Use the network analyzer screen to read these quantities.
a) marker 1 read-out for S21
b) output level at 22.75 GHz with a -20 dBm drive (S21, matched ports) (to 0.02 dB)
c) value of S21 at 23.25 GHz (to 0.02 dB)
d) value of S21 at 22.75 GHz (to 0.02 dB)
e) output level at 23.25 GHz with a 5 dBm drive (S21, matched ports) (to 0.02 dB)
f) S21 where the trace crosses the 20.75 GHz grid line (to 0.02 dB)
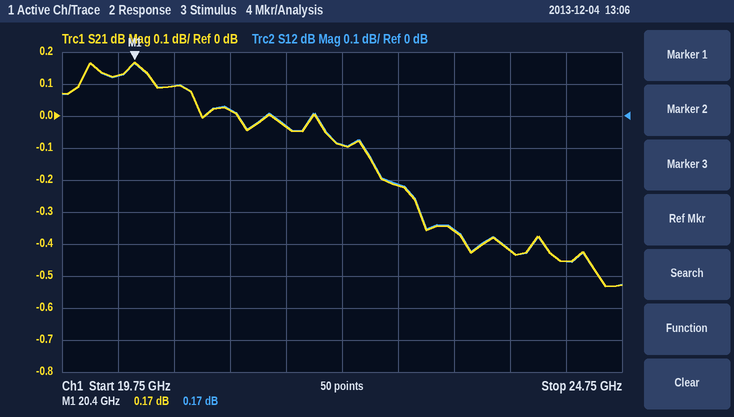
0.17 dB
-20.22 dBm
-0.36 dB
-0.22 dB
4.64 dBm
0.10 dB
